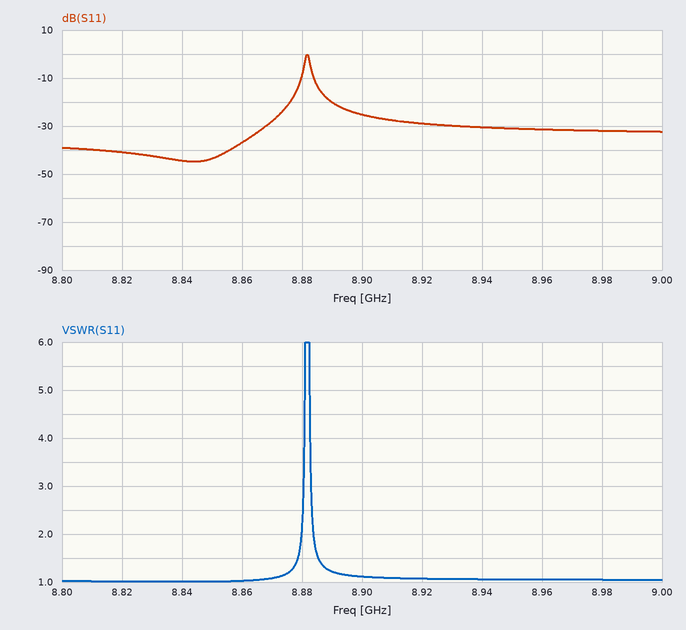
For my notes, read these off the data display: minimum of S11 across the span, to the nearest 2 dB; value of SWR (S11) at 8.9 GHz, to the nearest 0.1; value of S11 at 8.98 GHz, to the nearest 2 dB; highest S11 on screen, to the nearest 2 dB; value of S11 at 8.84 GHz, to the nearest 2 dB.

-44 dB
1.1
-32 dB
0 dB
-44 dB
